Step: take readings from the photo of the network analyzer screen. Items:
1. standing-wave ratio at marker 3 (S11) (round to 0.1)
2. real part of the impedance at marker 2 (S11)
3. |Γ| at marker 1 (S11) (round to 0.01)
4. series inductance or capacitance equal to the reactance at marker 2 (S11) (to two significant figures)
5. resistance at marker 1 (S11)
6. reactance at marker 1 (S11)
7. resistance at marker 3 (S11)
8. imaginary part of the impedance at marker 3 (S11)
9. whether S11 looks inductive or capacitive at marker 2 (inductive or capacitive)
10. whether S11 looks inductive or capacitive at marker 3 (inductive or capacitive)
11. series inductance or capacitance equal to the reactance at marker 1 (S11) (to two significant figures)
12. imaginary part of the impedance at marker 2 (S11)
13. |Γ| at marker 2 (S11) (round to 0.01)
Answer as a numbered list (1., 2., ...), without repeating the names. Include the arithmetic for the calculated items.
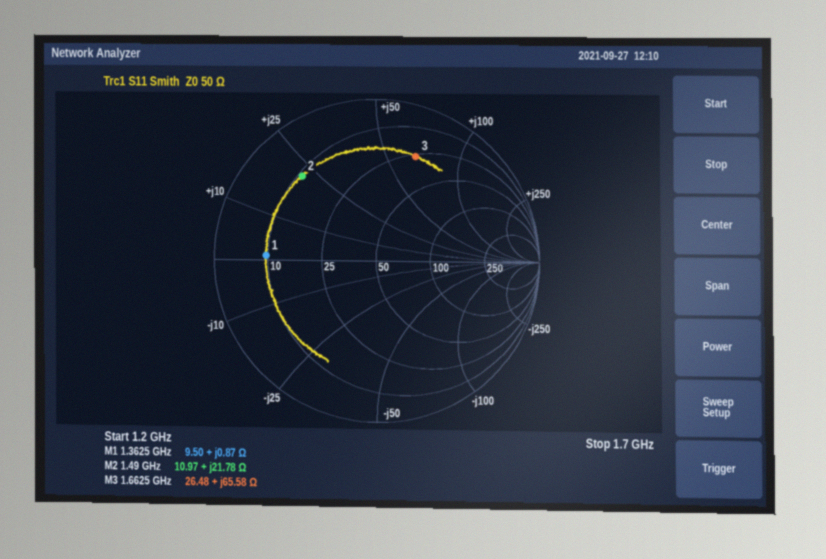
1. 5.5
2. 10.97 Ω
3. 0.68
4. L = 21.78 Ω/(2π × 1.49 GHz) ≈ 2.3 nH
5. 9.50 Ω
6. +0.87 Ω
7. 26.48 Ω
8. +65.58 Ω
9. inductive
10. inductive
11. L = 0.87 Ω/(2π × 1.3625 GHz) ≈ 102 pH, so 100 pH to two significant figures
12. +21.78 Ω
13. 0.69
